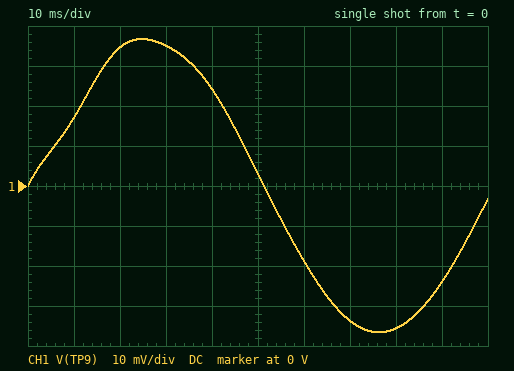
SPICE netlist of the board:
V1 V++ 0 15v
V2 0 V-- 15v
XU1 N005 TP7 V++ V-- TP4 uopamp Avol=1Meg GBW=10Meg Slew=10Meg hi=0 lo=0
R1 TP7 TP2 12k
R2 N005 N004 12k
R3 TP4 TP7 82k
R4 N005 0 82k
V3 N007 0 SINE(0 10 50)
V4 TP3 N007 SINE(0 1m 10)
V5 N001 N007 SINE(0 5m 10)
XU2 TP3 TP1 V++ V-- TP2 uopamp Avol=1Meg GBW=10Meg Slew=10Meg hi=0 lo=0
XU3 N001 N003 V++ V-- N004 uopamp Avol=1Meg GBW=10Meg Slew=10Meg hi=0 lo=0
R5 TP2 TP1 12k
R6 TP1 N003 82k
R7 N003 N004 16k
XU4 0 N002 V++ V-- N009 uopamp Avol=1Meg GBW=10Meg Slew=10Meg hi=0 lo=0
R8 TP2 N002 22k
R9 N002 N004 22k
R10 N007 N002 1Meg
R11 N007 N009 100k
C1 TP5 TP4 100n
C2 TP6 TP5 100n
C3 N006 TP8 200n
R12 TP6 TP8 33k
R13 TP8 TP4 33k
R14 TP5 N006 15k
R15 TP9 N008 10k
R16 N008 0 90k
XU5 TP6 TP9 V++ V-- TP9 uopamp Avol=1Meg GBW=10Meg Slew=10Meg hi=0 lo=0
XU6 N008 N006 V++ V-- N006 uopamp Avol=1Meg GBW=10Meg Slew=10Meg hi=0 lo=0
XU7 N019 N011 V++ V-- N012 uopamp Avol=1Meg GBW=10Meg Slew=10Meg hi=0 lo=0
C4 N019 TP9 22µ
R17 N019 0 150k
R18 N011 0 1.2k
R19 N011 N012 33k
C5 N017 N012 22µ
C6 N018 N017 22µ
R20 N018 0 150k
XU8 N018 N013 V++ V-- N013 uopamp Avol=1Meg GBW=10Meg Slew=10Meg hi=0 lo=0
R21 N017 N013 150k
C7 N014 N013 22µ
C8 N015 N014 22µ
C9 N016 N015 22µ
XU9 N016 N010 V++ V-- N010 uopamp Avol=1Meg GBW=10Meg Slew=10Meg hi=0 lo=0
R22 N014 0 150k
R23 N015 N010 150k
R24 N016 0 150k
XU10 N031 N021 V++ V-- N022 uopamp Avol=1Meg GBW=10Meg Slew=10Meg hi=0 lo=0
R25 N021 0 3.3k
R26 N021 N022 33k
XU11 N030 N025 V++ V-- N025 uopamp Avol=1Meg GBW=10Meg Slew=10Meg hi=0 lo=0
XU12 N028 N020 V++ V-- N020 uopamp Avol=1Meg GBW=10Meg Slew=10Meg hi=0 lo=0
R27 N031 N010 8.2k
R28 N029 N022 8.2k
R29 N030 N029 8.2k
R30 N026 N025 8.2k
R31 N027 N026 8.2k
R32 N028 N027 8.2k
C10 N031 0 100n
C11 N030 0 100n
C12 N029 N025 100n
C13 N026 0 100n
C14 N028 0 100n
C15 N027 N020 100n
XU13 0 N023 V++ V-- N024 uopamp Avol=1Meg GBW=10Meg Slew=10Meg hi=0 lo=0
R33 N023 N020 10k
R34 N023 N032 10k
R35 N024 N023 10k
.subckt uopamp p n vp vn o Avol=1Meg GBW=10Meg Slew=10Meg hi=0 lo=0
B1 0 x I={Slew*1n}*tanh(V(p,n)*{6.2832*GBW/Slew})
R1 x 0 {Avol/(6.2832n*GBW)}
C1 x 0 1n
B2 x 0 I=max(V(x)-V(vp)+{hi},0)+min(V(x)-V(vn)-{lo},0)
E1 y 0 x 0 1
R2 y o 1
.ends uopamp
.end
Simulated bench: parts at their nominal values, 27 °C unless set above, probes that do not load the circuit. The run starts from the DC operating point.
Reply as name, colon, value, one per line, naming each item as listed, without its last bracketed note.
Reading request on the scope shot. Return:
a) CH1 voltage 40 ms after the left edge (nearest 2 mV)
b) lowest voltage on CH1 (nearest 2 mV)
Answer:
CH1 voltage 40 ms after the left edge: 24 mV
lowest voltage on CH1: -36 mV
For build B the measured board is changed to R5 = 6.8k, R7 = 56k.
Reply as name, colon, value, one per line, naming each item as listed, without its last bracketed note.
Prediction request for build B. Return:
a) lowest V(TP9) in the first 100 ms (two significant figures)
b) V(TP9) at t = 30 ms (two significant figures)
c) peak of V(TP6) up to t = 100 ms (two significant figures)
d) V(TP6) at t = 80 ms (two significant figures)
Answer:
lowest V(TP9) in the first 100 ms: -48 mV
V(TP9) at t = 30 ms: 46 mV
peak of V(TP6) up to t = 100 ms: 48 mV
V(TP6) at t = 80 ms: -47 mV
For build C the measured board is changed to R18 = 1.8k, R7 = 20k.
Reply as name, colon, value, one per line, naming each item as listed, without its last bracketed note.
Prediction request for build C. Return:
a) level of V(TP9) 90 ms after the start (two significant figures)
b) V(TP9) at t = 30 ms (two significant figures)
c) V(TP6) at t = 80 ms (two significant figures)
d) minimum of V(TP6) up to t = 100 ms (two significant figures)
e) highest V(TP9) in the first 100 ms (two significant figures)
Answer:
level of V(TP9) 90 ms after the start: -25 mV
V(TP9) at t = 30 ms: 36 mV
V(TP6) at t = 80 ms: -37 mV
minimum of V(TP6) up to t = 100 ms: -38 mV
highest V(TP9) in the first 100 ms: 38 mV
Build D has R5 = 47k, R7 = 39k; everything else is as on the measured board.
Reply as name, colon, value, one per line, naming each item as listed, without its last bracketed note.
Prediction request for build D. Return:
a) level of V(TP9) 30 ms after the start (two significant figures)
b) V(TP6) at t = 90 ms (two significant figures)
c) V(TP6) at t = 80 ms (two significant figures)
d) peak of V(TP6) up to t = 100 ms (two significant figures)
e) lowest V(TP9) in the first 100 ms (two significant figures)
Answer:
level of V(TP9) 30 ms after the start: 54 mV
V(TP6) at t = 90 ms: -37 mV
V(TP6) at t = 80 ms: -54 mV
peak of V(TP6) up to t = 100 ms: 56 mV
lowest V(TP9) in the first 100 ms: -56 mV
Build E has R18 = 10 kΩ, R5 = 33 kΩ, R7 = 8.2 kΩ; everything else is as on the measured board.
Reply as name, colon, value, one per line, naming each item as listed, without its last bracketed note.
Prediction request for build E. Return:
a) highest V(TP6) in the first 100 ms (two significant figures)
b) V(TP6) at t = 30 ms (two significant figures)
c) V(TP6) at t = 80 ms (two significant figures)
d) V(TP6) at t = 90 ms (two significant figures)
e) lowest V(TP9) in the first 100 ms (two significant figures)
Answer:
highest V(TP6) in the first 100 ms: 41 mV
V(TP6) at t = 30 ms: 39 mV
V(TP6) at t = 80 ms: -40 mV
V(TP6) at t = 90 ms: -27 mV
lowest V(TP9) in the first 100 ms: -41 mV
